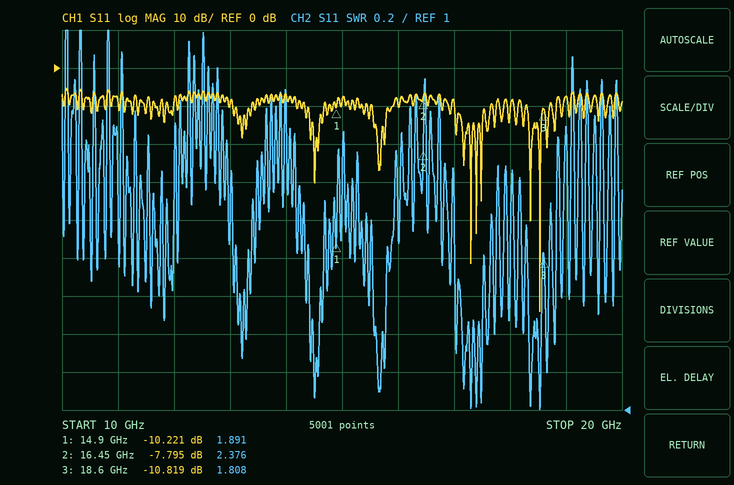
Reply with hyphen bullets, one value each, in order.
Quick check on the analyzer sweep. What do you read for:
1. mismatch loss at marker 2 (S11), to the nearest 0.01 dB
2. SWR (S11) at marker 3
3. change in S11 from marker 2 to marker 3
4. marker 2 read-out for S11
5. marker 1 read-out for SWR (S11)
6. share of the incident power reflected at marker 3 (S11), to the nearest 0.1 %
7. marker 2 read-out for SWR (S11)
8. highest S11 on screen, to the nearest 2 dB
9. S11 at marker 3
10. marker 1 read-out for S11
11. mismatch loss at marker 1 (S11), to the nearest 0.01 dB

- 0.79 dB
- 1.808
- -3.024 dB
- -7.795 dB
- 1.891
- 8.3 %
- 2.376
- -6 dB
- -10.819 dB
- -10.221 dB
- 0.43 dB
